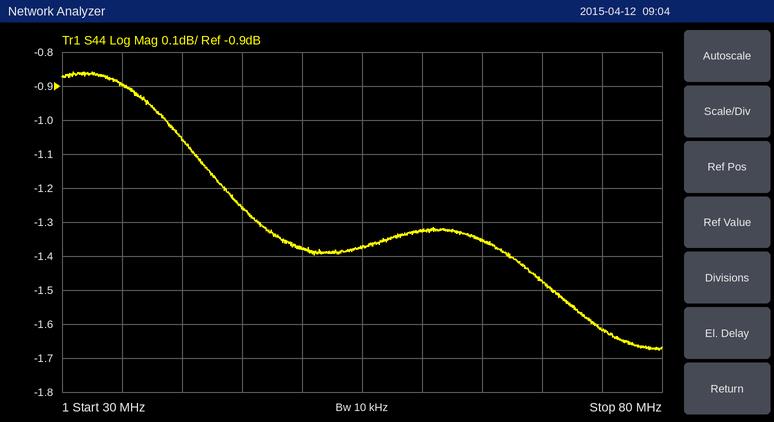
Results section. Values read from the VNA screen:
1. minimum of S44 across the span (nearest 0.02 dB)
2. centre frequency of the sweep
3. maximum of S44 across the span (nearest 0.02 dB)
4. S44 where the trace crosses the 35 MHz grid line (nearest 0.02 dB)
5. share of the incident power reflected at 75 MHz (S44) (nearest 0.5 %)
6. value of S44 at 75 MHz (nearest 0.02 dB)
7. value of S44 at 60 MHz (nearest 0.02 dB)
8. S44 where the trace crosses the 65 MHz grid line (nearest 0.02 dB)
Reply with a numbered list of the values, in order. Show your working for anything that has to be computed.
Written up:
1. -1.68 dB
2. 55 MHz
3. -0.86 dB
4. -0.90 dB
5. 10^(-1.62/10) ≈ 68.9 %, so 69.0 % to the nearest 0.5 %
6. -1.62 dB
7. -1.32 dB
8. -1.36 dB
